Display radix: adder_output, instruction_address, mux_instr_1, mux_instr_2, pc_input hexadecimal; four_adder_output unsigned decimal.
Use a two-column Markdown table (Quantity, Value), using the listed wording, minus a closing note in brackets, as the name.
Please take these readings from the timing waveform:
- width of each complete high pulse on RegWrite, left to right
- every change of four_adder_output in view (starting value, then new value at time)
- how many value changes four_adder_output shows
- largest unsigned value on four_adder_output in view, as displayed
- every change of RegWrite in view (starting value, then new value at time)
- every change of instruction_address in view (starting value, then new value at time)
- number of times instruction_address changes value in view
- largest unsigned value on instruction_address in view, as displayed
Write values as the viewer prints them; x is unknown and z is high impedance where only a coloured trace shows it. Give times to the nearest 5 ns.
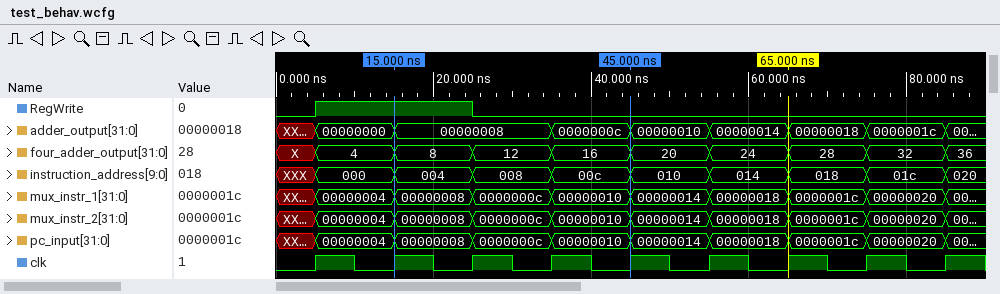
| Quantity | Value |
|---|---|
| width of each complete high pulse on RegWrite, left to right | 20 ns |
| every change of four_adder_output in view | X, 4 at 5 ns, 8 at 15 ns, 12 at 25 ns, 16 at 35 ns, 20 at 45 ns, 24 at 55 ns, 28 at 65 ns, 32 at 75 ns, 36 at 85 ns |
| how many value changes four_adder_output shows | 9 |
| largest unsigned value on four_adder_output in view, as displayed | 36 |
| every change of RegWrite in view | 0, 1 at 5 ns, 0 at 25 ns |
| every change of instruction_address in view | XXX, 000 at 5 ns, 004 at 15 ns, 008 at 25 ns, 00c at 35 ns, 010 at 45 ns, 014 at 55 ns, 018 at 65 ns, 01c at 75 ns, 020 at 85 ns |
| number of times instruction_address changes value in view | 9 |
| largest unsigned value on instruction_address in view, as displayed | 020 |
